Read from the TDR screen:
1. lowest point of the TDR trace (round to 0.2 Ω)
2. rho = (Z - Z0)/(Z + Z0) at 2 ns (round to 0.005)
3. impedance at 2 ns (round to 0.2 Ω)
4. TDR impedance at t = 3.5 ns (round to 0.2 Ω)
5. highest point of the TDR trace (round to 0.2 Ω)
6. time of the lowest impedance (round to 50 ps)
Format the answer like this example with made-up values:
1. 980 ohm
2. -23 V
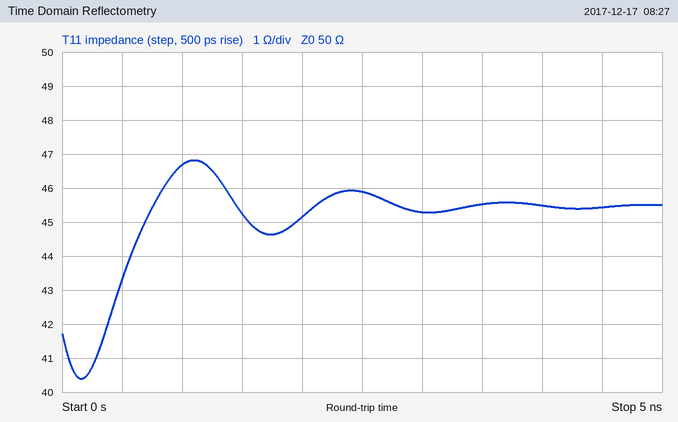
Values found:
1. 40.4 Ω
2. -0.050
3. 45.2 Ω
4. 45.6 Ω
5. 46.8 Ω
6. 150 ps
